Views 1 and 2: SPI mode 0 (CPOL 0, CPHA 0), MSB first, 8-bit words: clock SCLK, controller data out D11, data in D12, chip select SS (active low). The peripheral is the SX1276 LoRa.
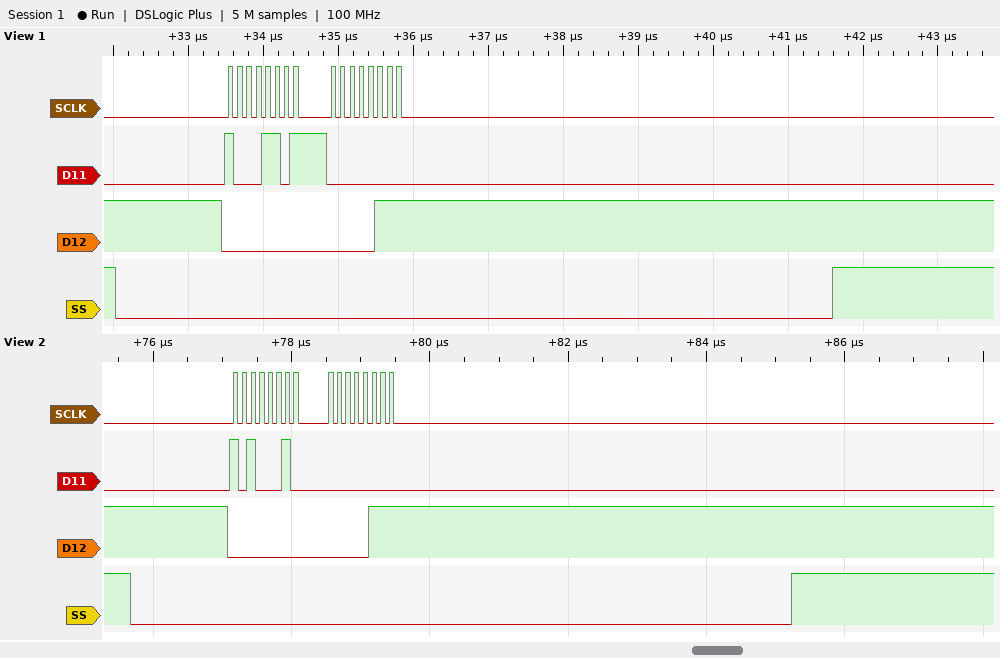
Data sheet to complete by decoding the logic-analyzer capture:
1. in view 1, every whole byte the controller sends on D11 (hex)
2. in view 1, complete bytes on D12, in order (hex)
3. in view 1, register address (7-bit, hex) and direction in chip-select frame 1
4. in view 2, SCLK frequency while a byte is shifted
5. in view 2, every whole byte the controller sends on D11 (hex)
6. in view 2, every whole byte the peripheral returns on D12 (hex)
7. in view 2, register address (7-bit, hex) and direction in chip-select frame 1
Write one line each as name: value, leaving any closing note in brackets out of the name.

in view 1, every whole byte the controller sends on D11: 0x8D 0x00
in view 1, complete bytes on D12, in order: 0x00 0x07
in view 1, register address (7-bit, hex) and direction in chip-select frame 1: 0x0D write
in view 2, SCLK frequency while a byte is shifted: 8 MHz
in view 2, every whole byte the controller sends on D11: A2 00
in view 2, every whole byte the peripheral returns on D12: 00 07
in view 2, register address (7-bit, hex) and direction in chip-select frame 1: 0x22 write
